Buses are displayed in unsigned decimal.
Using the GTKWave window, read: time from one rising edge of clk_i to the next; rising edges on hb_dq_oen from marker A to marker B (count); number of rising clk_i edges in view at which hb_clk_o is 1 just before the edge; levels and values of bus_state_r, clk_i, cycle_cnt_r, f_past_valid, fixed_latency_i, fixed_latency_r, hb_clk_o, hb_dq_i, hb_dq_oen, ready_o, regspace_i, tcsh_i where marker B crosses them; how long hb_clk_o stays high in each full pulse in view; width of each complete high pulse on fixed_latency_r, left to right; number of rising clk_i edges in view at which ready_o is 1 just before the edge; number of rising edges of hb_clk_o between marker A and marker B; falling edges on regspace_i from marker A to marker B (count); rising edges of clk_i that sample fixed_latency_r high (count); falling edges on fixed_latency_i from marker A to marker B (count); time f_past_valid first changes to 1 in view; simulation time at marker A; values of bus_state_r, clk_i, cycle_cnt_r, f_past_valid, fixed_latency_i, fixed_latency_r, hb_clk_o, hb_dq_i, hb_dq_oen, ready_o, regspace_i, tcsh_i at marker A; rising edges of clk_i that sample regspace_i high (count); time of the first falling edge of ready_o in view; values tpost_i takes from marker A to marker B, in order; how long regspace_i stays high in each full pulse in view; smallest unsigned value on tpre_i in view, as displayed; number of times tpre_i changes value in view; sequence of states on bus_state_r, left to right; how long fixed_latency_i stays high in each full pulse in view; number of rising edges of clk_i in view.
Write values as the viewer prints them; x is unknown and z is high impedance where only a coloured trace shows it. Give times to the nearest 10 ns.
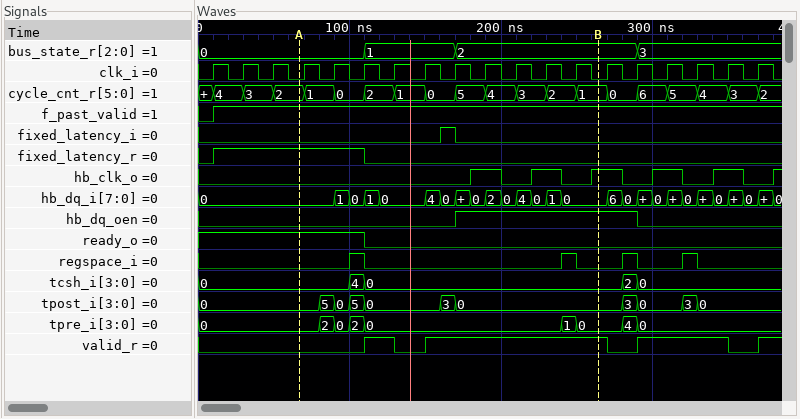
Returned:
20 ns
1
5
bus_state_r=2, clk_i=0, cycle_cnt_r=1, f_past_valid=1, fixed_latency_i=0, fixed_latency_r=0, hb_clk_o=1, hb_dq_i=0, hb_dq_oen=1, ready_o=0, regspace_i=0, tcsh_i=0
20 ns, 20 ns, 20 ns, 20 ns, 20 ns
100 ns
6
3
2
5
1
10 ns
70 ns
bus_state_r=0, clk_i=0, cycle_cnt_r=2, f_past_valid=1, fixed_latency_i=0, fixed_latency_r=1, hb_clk_o=0, hb_dq_i=0, hb_dq_oen=0, ready_o=1, regspace_i=0, tcsh_i=0
4
110 ns
0, 5, 0, 5, 0, 3, 0
10 ns, 10 ns, 10 ns, 10 ns
0
8
0, 1, 2, 3
10 ns
19
